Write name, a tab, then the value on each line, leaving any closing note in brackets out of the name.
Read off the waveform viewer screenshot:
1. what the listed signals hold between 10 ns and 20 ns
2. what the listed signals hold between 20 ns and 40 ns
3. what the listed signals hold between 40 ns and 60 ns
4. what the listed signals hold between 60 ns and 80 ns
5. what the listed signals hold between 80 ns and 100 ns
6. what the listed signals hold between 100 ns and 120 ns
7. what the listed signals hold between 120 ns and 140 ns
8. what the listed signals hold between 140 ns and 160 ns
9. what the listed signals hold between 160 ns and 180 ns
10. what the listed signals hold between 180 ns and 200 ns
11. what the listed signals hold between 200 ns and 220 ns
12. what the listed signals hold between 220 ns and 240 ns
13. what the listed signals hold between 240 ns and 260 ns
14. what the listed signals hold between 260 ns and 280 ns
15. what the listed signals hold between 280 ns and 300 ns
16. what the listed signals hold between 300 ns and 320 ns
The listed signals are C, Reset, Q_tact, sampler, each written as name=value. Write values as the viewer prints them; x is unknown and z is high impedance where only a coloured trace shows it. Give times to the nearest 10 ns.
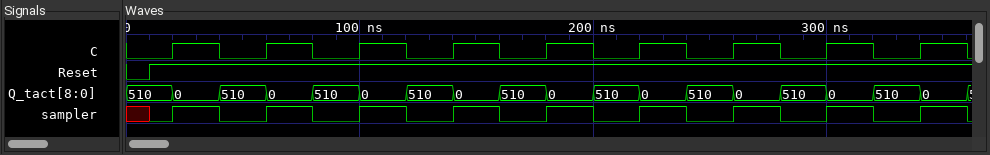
what the listed signals hold between 10 ns and 20 ns	C=0, Reset=1, Q_tact=510, sampler=0
what the listed signals hold between 20 ns and 40 ns	C=1, Reset=1, Q_tact=0, sampler=1
what the listed signals hold between 40 ns and 60 ns	C=0, Reset=1, Q_tact=510, sampler=0
what the listed signals hold between 60 ns and 80 ns	C=1, Reset=1, Q_tact=0, sampler=1
what the listed signals hold between 80 ns and 100 ns	C=0, Reset=1, Q_tact=510, sampler=0
what the listed signals hold between 100 ns and 120 ns	C=1, Reset=1, Q_tact=0, sampler=1
what the listed signals hold between 120 ns and 140 ns	C=0, Reset=1, Q_tact=510, sampler=0
what the listed signals hold between 140 ns and 160 ns	C=1, Reset=1, Q_tact=0, sampler=1
what the listed signals hold between 160 ns and 180 ns	C=0, Reset=1, Q_tact=510, sampler=0
what the listed signals hold between 180 ns and 200 ns	C=1, Reset=1, Q_tact=0, sampler=1
what the listed signals hold between 200 ns and 220 ns	C=0, Reset=1, Q_tact=510, sampler=0
what the listed signals hold between 220 ns and 240 ns	C=1, Reset=1, Q_tact=0, sampler=1
what the listed signals hold between 240 ns and 260 ns	C=0, Reset=1, Q_tact=510, sampler=0
what the listed signals hold between 260 ns and 280 ns	C=1, Reset=1, Q_tact=0, sampler=1
what the listed signals hold between 280 ns and 300 ns	C=0, Reset=1, Q_tact=510, sampler=0
what the listed signals hold between 300 ns and 320 ns	C=1, Reset=1, Q_tact=0, sampler=1
